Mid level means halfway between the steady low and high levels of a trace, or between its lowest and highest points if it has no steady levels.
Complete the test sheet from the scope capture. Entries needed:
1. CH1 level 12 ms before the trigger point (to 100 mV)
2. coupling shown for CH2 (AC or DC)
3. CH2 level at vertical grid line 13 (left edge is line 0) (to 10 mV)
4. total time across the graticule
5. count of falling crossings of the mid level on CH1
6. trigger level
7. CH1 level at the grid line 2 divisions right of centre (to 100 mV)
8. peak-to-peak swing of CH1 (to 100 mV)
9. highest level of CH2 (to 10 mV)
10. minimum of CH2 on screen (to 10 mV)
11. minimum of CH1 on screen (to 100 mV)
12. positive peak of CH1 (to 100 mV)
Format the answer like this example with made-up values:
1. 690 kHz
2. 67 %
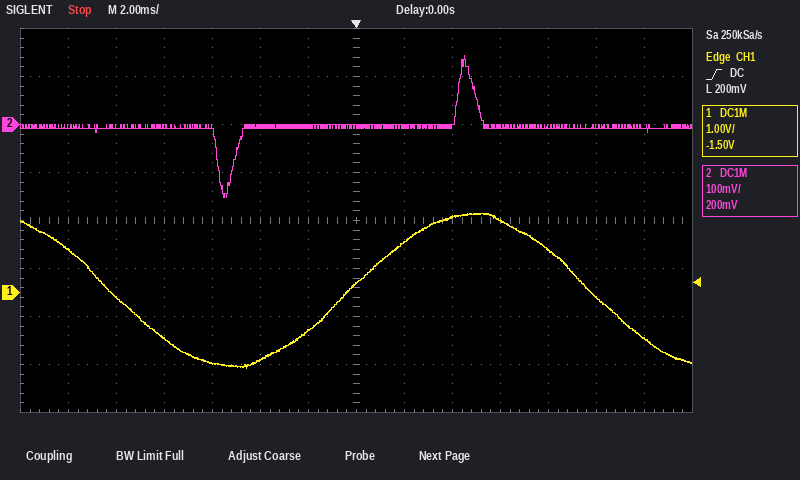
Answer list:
1. 900 mV
2. DC
3. -10 mV
4. 28 ms
5. 2
6. 200 mV
7. 1.6 V
8. 3.2 V
9. 140 mV
10. -150 mV
11. -1.6 V
12. 1.6 V
